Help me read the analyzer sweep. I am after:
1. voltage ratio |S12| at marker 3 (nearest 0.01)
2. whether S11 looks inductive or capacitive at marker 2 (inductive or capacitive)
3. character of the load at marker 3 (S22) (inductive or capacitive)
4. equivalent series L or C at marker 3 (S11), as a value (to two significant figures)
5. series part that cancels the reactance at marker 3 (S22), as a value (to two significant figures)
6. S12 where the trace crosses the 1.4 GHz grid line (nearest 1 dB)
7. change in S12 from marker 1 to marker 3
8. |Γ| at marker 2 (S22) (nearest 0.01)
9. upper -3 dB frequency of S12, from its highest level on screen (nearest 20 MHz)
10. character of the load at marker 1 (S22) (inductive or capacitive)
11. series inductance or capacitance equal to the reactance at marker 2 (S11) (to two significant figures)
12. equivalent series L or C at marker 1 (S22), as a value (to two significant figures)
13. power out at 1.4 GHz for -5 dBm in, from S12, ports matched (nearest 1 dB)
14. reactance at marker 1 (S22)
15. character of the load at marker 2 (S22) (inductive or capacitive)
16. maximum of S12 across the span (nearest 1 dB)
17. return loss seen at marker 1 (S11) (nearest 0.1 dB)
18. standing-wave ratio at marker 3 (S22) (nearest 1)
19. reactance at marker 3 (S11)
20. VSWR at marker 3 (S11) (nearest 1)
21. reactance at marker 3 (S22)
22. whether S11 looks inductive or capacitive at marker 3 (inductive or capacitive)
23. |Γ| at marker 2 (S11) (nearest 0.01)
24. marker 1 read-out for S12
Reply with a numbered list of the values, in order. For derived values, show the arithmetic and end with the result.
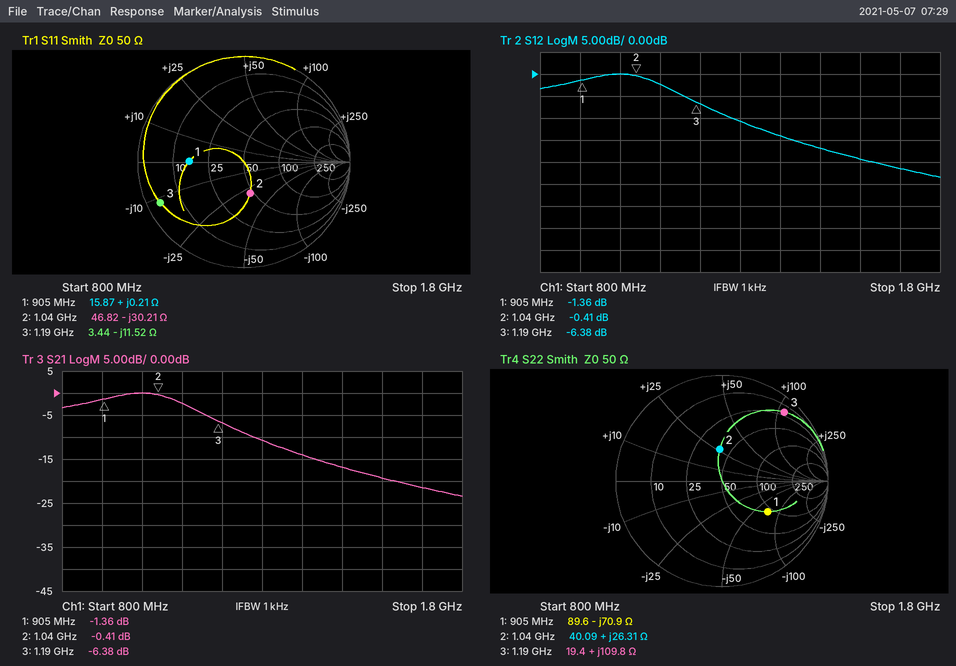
1. 10^(-6.38/20) ≈ 0.48
2. capacitive
3. inductive
4. C = 1/(2π × 1.19 GHz × 11.52 Ω) ≈ 12 pF
5. C = 1/(2π × 1.19 GHz × 109.8 Ω) ≈ 1.2 pF
6. -14 dB
7. -6.38 − (-1.36) = -5.02 dB
8. 0.30
9. 1.12 GHz
10. capacitive
11. C = 1/(2π × 1.04 GHz × 30.21 Ω) ≈ 5.1 pF
12. C = 1/(2π × 905 MHz × 70.9 Ω) ≈ 2.5 pF
13. -5 dBm + (-14 dB) = -19 dBm
14. -70.9 Ω
15. inductive
16. 0 dB
17. 5.7 dB
18. 15
19. -11.52 Ω
20. 15
21. +109.8 Ω
22. capacitive
23. 0.30
24. -1.36 dB
